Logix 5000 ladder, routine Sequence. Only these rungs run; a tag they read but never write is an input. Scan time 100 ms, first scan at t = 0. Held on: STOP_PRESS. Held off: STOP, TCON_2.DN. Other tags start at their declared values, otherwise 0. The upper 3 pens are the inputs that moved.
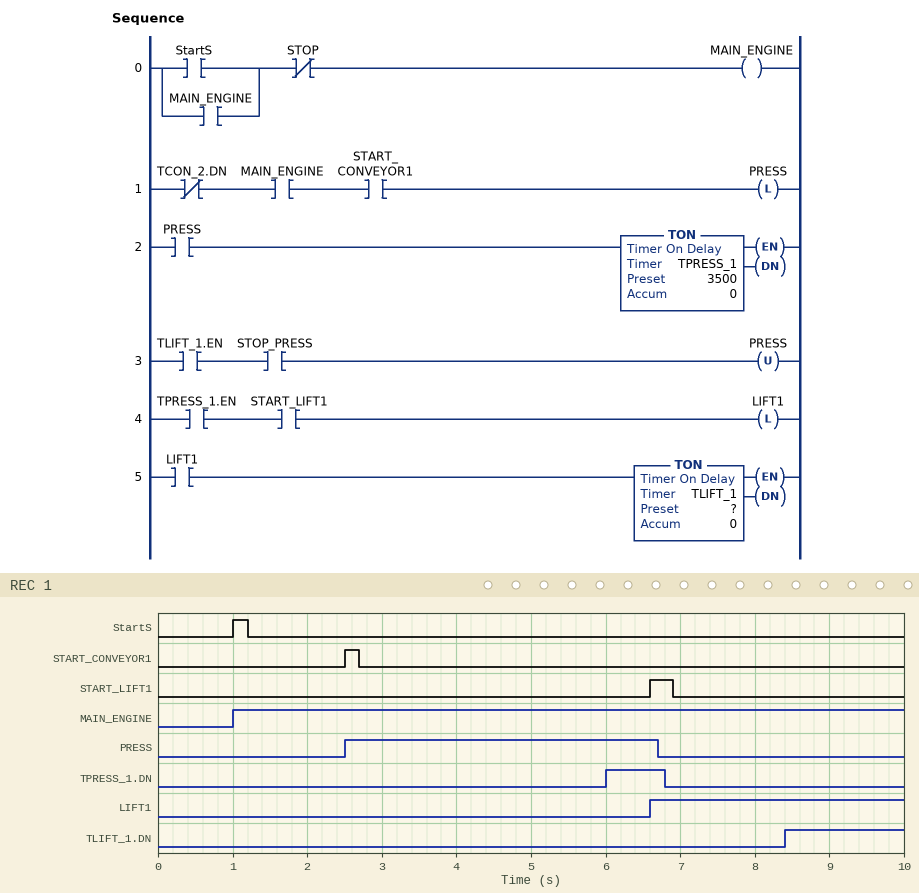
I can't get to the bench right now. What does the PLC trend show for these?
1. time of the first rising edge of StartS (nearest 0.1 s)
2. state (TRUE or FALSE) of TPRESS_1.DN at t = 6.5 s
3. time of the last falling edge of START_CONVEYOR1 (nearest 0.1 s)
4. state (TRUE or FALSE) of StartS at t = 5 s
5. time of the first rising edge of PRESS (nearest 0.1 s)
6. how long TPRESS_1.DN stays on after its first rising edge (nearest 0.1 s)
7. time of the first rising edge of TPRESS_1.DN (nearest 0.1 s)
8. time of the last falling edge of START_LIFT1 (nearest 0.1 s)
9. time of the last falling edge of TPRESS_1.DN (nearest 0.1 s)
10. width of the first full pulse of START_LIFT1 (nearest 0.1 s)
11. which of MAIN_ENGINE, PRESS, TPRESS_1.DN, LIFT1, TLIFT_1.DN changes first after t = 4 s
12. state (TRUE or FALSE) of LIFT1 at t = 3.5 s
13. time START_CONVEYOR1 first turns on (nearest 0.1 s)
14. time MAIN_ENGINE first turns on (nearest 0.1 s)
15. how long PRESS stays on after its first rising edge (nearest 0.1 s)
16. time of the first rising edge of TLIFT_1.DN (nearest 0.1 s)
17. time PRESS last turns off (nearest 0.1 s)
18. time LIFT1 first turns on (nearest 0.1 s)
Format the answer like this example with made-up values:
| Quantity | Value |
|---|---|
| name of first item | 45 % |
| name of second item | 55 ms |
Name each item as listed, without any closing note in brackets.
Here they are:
| Quantity | Value |
|---|---|
| time of the first rising edge of StartS | 1.0 s |
| state (TRUE or FALSE) of TPRESS_1.DN at t = 6.5 s | TRUE |
| time of the last falling edge of START_CONVEYOR1 | 2.7 s |
| state (TRUE or FALSE) of StartS at t = 5 s | FALSE |
| time of the first rising edge of PRESS | 2.5 s |
| how long TPRESS_1.DN stays on after its first rising edge | 0.8 s |
| time of the first rising edge of TPRESS_1.DN | 6.0 s |
| time of the last falling edge of START_LIFT1 | 6.9 s |
| time of the last falling edge of TPRESS_1.DN | 6.8 s |
| width of the first full pulse of START_LIFT1 | 0.3 s |
| which of MAIN_ENGINE, PRESS, TPRESS_1.DN, LIFT1, TLIFT_1.DN changes first after t = 4 s | TPRESS_1.DN |
| state (TRUE or FALSE) of LIFT1 at t = 3.5 s | FALSE |
| time START_CONVEYOR1 first turns on | 2.5 s |
| time MAIN_ENGINE first turns on | 1.0 s |
| how long PRESS stays on after its first rising edge | 4.2 s |
| time of the first rising edge of TLIFT_1.DN | 8.4 s |
| time PRESS last turns off | 6.7 s |
| time LIFT1 first turns on | 6.6 s |
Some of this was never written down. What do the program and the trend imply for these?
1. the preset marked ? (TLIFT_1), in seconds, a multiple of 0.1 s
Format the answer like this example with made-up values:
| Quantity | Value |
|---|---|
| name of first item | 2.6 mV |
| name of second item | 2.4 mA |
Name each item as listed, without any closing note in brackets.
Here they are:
| Quantity | Value |
|---|---|
| the preset marked ? (TLIFT_1), in seconds, a multiple of 0.1 s | 1.8 s |
